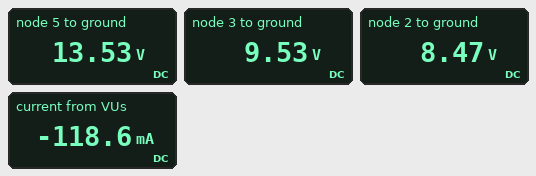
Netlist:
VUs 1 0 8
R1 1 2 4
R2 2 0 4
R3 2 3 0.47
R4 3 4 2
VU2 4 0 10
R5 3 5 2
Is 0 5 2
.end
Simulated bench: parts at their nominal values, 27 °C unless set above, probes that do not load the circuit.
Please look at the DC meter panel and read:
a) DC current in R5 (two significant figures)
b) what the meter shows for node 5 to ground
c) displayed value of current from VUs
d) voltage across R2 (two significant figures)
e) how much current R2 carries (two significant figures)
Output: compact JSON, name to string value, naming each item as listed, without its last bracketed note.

{"DC current in R5": "2.0 A", "what the meter shows for node 5 to ground": "13.53 V", "displayed value of current from VUs": "-118.6 mA", "voltage across R2": "8.5 V", "how much current R2 carries": "2.1 A"}
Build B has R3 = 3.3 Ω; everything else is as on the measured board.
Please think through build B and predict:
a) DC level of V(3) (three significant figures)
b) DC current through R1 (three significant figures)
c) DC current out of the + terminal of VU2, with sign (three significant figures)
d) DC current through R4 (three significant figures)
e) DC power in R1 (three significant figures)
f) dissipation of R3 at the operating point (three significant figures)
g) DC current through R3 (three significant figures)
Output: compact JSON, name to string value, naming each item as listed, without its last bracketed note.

{"DC level of V(3)": "11.3 V", "DC current through R1": "315 mA", "DC current out of the + terminal of VU2, with sign": "-630 mA", "DC current through R4": "630 mA", "DC power in R1": "397 mW", "dissipation of R3 at the operating point": "6.19 W", "DC current through R3": "1.37 A"}
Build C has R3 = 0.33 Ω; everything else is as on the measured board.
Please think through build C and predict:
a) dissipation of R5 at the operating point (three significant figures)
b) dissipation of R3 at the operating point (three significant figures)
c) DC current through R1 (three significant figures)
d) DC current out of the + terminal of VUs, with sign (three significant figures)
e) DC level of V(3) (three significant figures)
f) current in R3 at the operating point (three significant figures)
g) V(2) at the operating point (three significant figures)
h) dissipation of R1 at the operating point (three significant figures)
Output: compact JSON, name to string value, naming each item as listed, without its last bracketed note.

{"dissipation of R5 at the operating point": "8.00 W", "dissipation of R3 at the operating point": "1.76 W", "DC current through R1": "155 mA", "DC current out of the + terminal of VUs, with sign": "-155 mA", "DC level of V(3)": "9.38 V", "current in R3 at the operating point": "2.31 A", "V(2) at the operating point": "8.62 V", "dissipation of R1 at the operating point": "95.8 mW"}
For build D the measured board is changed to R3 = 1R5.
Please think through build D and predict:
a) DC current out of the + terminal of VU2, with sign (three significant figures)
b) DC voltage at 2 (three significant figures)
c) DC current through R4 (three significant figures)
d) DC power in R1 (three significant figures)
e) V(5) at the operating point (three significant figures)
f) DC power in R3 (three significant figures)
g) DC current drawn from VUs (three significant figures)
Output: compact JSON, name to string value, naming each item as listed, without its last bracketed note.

{"DC current out of the + terminal of VU2, with sign": "-182 mA", "DC voltage at 2": "7.64 V", "DC current through R4": "182 mA", "DC power in R1": "33.1 mW", "V(5) at the operating point": "14.4 V", "DC power in R3": "4.96 W", "DC current drawn from VUs": "90.9 mA"}
